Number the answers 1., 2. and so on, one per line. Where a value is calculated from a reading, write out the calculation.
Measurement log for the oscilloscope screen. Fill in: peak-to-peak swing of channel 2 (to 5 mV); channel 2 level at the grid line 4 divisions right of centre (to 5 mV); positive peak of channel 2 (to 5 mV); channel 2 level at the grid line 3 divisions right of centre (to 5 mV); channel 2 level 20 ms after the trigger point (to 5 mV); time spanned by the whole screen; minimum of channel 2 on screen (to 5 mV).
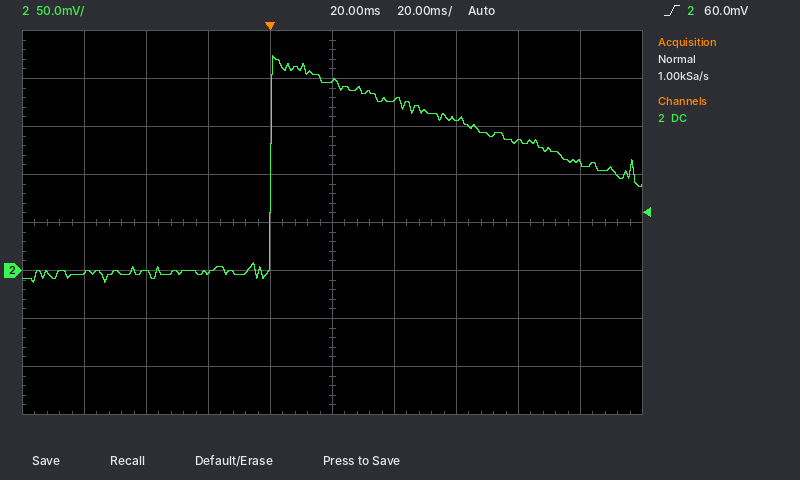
1. 225 mV − (-10 mV) = 235 mV
2. 110 mV
3. 225 mV
4. 135 mV
5. 200 mV
6. 200 ms
7. -10 mV
